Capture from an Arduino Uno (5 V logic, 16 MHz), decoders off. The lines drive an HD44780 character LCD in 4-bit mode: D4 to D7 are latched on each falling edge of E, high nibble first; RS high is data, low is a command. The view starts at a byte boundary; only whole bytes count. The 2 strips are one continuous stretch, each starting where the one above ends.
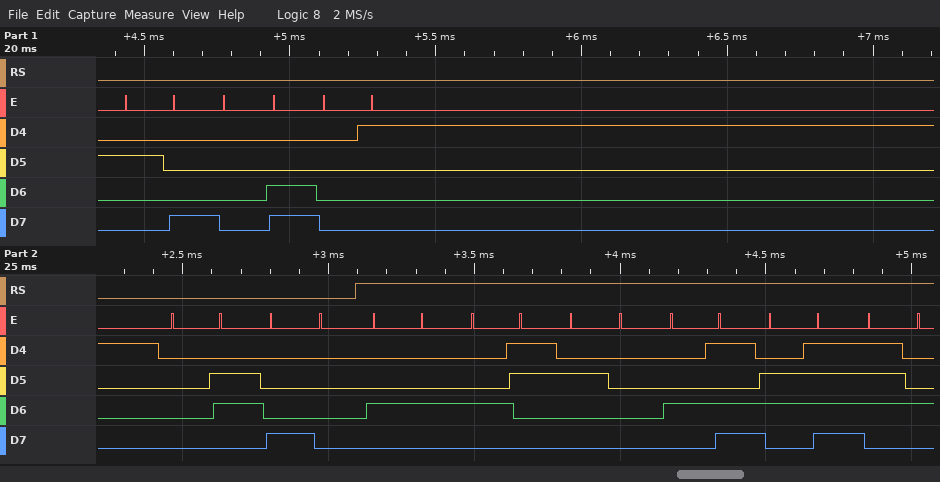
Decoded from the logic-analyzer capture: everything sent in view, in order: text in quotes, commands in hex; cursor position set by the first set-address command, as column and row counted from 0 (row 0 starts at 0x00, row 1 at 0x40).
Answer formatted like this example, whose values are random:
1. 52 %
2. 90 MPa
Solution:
1. 0x28 0x0C 0x01 0x06 0x80 "DC Mot"
2. column 0, row 0
